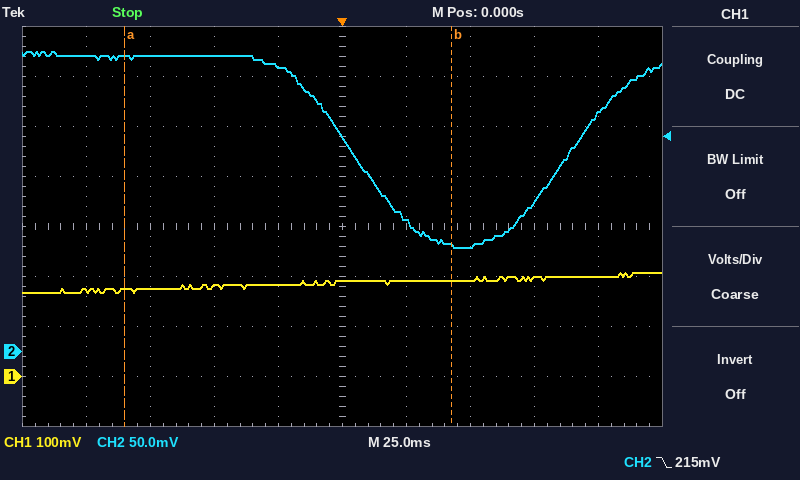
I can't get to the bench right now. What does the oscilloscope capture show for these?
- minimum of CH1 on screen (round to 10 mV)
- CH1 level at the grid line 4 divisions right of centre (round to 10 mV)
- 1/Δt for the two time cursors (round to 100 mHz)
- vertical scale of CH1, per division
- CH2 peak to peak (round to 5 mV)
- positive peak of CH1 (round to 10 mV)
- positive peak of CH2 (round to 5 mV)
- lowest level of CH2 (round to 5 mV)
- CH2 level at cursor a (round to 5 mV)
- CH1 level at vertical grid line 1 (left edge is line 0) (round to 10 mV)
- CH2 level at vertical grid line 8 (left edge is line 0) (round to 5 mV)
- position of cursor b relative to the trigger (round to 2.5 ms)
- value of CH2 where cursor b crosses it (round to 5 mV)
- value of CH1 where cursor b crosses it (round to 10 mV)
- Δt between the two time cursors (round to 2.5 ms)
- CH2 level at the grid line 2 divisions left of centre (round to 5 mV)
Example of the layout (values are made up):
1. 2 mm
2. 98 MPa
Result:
1. 170 mV
2. 200 mV
3. 7.8 Hz
4. 100 mV
5. 195 mV
6. 210 mV
7. 300 mV
8. 105 mV
9. 295 mV
10. 170 mV
11. 150 mV
12. +42.5 ms
13. 105 mV
14. 190 mV
15. 127.5 ms
16. 295 mV
